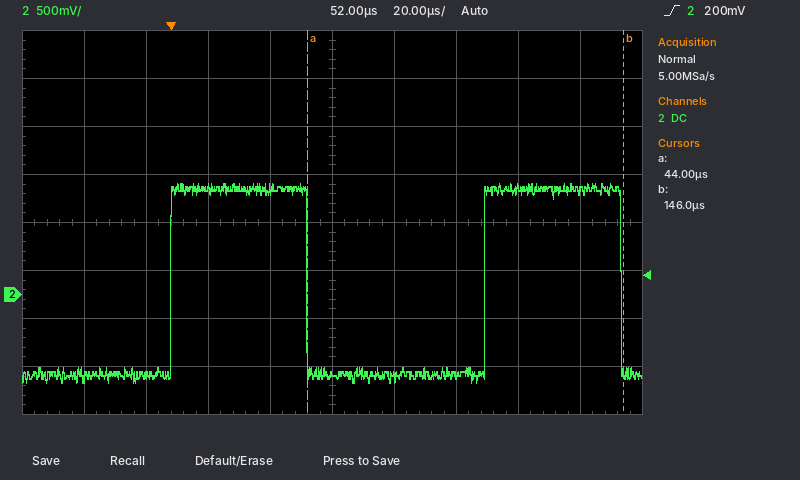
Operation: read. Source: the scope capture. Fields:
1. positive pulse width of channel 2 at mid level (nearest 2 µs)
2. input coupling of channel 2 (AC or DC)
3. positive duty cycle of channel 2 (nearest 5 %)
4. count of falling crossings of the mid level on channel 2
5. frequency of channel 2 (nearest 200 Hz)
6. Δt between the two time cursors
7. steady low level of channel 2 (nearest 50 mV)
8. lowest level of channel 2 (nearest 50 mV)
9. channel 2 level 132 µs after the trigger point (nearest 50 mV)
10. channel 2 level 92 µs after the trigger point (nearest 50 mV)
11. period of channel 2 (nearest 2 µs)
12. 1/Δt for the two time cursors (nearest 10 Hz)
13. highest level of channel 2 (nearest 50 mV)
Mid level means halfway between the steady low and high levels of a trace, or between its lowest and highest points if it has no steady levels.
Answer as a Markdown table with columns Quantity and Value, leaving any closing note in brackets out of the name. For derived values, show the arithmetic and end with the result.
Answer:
| Quantity | Value |
|---|---|
| positive pulse width of channel 2 at mid level | 44 µs |
| input coupling of channel 2 | DC |
| positive duty cycle of channel 2 | 44 µs / 102 µs ≈ 43.1 %, so 45 % to the nearest 5 % |
| count of falling crossings of the mid level on channel 2 | 2 |
| frequency of channel 2 | 1 / 102 µs ≈ 9.8 kHz |
| Δt between the two time cursors | 146 µs − (44 µs) = 102 µs |
| steady low level of channel 2 | -850 mV |
| lowest level of channel 2 | -900 mV |
| channel 2 level 132 µs after the trigger point | 1.10 V |
| channel 2 level 92 µs after the trigger point | -850 mV |
| period of channel 2 | 102 µs |
| 1/Δt for the two time cursors | 1 / 102 µs ≈ 9.80 kHz |
| highest level of channel 2 | 1.15 V |
